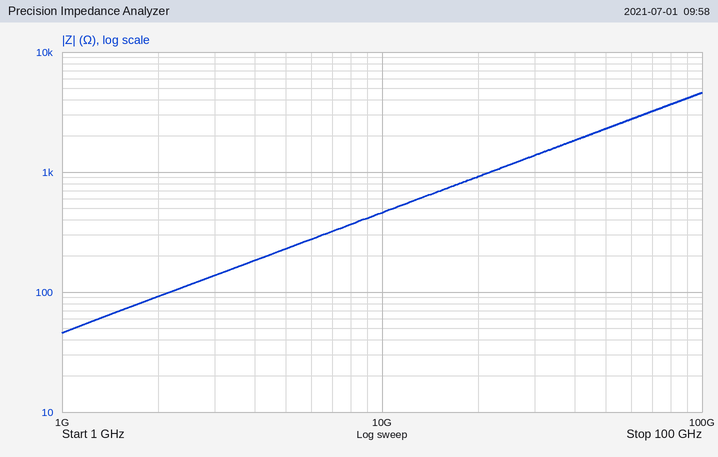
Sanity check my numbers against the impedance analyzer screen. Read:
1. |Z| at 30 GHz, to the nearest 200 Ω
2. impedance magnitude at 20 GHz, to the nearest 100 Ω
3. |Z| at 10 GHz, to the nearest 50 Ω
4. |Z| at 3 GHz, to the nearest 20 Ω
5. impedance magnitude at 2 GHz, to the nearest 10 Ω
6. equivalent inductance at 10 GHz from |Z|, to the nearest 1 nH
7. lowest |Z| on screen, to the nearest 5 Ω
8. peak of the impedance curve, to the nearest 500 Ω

1.4 kΩ
900 Ω
450 Ω
140 Ω
90 Ω
7 nH
45 Ω
4.5 kΩ
